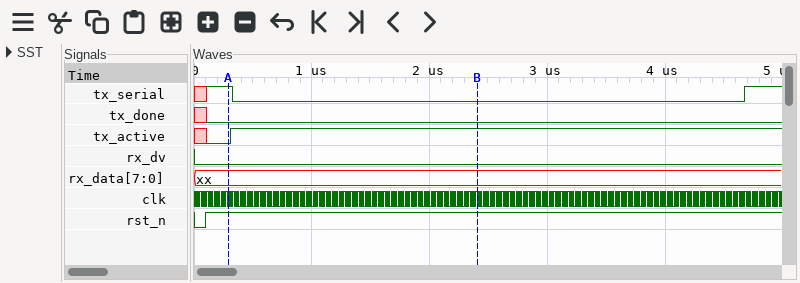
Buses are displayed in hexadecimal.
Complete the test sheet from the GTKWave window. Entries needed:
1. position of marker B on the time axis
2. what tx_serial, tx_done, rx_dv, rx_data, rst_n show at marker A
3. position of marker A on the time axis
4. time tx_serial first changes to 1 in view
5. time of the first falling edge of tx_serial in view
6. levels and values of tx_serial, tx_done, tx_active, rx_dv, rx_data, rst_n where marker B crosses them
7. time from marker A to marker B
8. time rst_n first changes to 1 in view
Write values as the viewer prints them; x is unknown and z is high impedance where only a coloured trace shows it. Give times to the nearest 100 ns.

2400 ns
tx_serial=1, tx_done=0, rx_dv=0, rx_data=xx, rst_n=1
300 ns
100 ns
300 ns
tx_serial=0, tx_done=0, tx_active=1, rx_dv=0, rx_data=xx, rst_n=1
2100 ns
100 ns
